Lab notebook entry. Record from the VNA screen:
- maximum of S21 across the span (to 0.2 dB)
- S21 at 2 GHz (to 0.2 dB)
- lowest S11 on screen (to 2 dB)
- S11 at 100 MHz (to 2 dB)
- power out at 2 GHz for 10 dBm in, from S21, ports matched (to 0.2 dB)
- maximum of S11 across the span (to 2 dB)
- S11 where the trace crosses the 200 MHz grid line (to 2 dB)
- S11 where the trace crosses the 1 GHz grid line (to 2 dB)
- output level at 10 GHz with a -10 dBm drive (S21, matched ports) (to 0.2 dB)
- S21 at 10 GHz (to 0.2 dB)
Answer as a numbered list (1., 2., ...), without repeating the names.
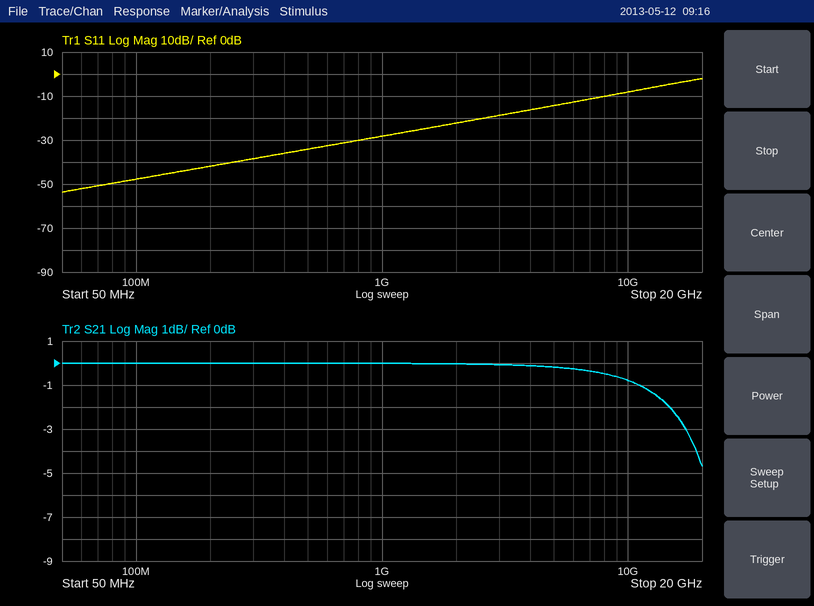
1. 0.0 dB
2. 0.0 dB
3. -54 dB
4. -48 dB
5. 10.0 dBm
6. -2 dB
7. -42 dB
8. -28 dB
9. -10.8 dBm
10. -0.8 dB
